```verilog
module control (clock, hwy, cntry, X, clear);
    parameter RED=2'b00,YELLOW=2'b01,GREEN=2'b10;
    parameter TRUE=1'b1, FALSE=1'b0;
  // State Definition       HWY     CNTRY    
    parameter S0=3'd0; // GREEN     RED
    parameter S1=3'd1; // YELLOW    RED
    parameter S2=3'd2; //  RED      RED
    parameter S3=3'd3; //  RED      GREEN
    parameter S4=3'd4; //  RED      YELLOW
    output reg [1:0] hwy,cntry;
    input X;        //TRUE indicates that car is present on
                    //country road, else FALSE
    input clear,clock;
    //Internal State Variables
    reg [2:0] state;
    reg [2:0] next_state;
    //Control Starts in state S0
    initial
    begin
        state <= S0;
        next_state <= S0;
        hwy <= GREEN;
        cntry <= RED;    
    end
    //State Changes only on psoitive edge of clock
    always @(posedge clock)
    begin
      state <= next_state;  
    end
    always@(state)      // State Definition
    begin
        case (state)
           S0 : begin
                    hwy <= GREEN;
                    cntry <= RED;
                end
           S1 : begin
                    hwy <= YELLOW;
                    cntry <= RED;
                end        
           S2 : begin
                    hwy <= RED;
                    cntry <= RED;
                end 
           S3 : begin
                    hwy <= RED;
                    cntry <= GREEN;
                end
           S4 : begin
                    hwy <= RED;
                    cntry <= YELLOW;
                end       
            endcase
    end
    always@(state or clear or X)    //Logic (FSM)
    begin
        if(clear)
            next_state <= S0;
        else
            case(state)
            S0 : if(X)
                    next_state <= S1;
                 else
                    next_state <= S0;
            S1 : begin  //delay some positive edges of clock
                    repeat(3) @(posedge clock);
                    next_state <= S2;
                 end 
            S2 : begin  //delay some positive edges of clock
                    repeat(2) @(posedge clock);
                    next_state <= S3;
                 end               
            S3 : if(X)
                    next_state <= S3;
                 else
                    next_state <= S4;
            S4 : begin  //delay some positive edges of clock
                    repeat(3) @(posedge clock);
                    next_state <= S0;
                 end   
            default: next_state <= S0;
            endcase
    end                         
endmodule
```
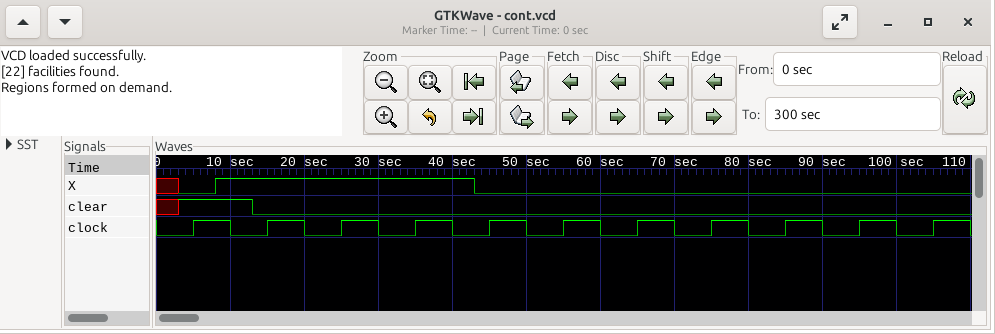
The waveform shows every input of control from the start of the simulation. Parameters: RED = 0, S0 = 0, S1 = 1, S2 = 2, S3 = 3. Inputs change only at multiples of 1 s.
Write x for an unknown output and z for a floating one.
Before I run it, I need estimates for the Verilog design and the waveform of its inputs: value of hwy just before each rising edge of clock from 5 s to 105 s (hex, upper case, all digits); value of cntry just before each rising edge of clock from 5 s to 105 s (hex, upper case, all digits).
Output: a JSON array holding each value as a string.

["2, 2, 1, 1, 1, 1, 0, 0, 0, 0, 0", "0, 0, 0, 0, 0, 0, 0, 0, 0, 2, 1"]
